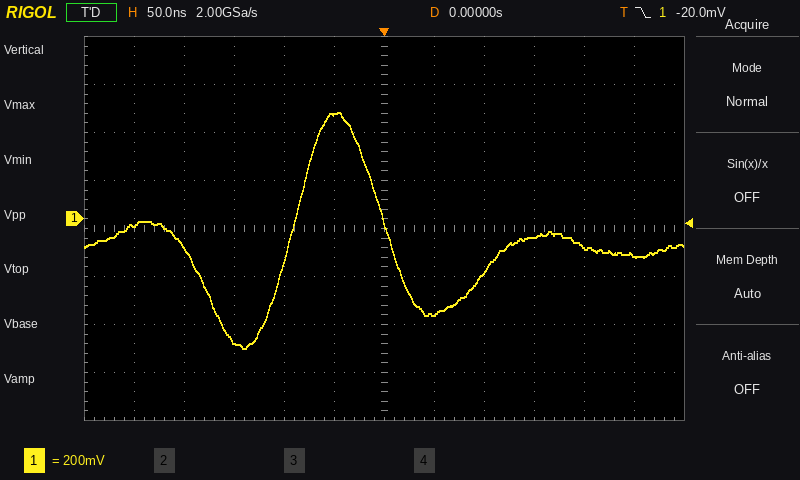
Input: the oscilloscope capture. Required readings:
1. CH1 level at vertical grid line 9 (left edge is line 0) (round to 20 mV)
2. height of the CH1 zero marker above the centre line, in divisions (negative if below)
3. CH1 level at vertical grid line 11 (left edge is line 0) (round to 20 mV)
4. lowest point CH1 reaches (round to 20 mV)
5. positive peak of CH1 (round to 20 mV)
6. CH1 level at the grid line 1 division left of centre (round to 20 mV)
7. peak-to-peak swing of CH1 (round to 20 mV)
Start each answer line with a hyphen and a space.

- -80 mV
- +0.2 div
- -160 mV
- -540 mV
- 440 mV
- 440 mV
- 980 mV
